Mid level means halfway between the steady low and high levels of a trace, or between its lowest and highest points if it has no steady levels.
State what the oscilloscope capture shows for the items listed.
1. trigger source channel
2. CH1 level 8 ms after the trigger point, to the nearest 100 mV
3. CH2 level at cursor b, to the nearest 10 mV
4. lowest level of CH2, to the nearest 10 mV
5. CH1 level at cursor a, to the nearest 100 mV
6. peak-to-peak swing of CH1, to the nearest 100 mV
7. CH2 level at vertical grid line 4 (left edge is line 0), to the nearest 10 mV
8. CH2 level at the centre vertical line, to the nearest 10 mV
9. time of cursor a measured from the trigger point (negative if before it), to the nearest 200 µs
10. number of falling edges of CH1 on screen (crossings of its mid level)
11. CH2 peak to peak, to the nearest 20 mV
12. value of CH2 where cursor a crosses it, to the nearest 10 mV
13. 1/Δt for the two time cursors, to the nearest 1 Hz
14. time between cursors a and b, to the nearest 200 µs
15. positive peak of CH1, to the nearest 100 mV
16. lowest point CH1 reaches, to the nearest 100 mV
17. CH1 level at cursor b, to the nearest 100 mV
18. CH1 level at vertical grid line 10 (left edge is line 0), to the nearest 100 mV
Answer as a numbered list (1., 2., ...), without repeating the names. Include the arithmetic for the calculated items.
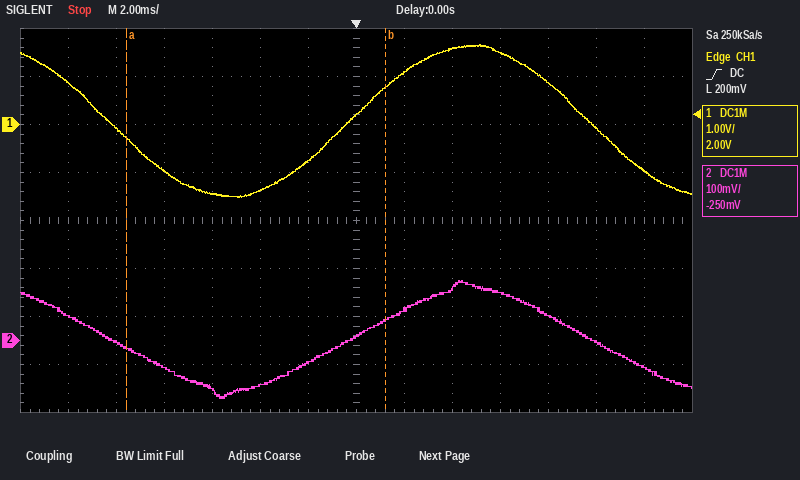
1. CH1
2. 900 mV
3. 40 mV
4. -120 mV
5. -300 mV
6. 1.7 V − (-1.5 V) = 3.2 V
7. -100 mV
8. 10 mV
9. -9.6 ms
10. 2
11. 240 mV
12. -20 mV
13. 1 / 10.8 ms ≈ 93 Hz
14. 10.8 ms
15. 1.7 V
16. -1.5 V
17. 800 mV
18. 1.5 V
